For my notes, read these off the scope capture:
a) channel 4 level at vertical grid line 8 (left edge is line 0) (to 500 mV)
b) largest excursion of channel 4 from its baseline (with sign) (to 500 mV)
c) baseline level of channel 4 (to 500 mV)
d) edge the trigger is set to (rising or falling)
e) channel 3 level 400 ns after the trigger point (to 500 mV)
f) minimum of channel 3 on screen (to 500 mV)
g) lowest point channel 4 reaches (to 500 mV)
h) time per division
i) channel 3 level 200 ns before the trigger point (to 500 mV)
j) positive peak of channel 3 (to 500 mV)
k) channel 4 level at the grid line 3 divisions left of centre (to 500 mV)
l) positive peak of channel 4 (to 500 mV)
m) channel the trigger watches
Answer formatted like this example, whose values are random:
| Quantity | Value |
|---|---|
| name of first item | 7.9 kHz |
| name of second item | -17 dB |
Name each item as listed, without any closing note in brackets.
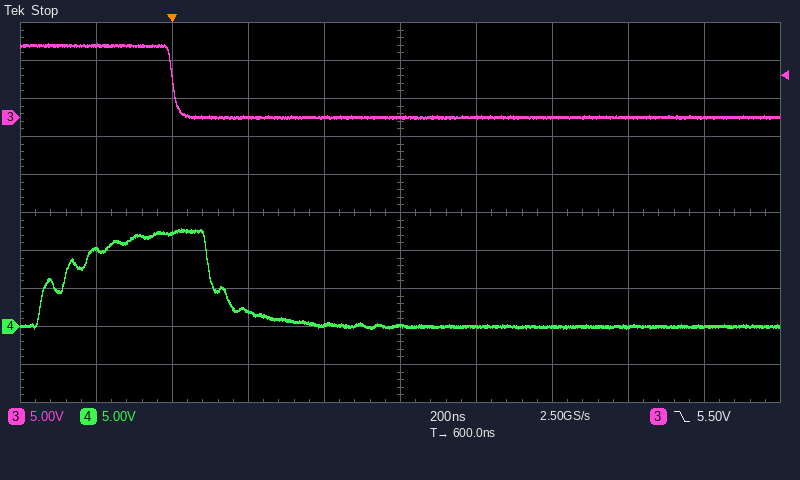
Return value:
| Quantity | Value |
|---|---|
| channel 4 level at vertical grid line 8 (left edge is line 0) | 0.0 V |
| largest excursion of channel 4 from its baseline (with sign) | +13.0 V |
| baseline level of channel 4 | 0.0 V |
| edge the trigger is set to | falling |
| channel 3 level 400 ns after the trigger point | 0.0 V |
| minimum of channel 3 on screen | 0.0 V |
| lowest point channel 4 reaches | -500 mV |
| time per division | 200 ns |
| channel 3 level 200 ns before the trigger point | 9.5 V |
| positive peak of channel 3 | 9.5 V |
| channel 4 level at the grid line 3 divisions left of centre | 12.5 V |
| positive peak of channel 4 | 13.0 V |
| channel the trigger watches | channel 3 |
